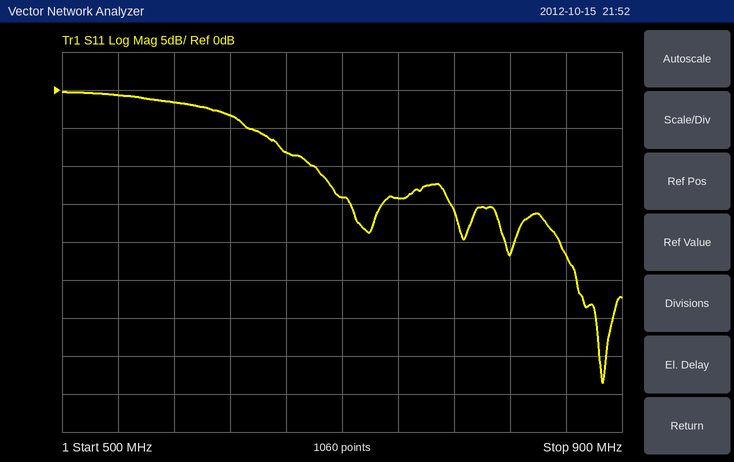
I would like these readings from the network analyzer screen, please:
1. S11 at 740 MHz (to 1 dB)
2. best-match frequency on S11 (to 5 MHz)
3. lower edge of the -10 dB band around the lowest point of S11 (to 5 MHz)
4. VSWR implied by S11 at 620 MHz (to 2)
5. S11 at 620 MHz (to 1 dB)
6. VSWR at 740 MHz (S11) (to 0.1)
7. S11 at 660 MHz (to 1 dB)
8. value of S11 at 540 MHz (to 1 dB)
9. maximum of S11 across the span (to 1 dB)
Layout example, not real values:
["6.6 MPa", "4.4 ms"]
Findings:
["-14 dB", "885 MHz", "680 MHz", "6", "-3 dB", "1.5", "-8 dB", "-1 dB", "0 dB"]
